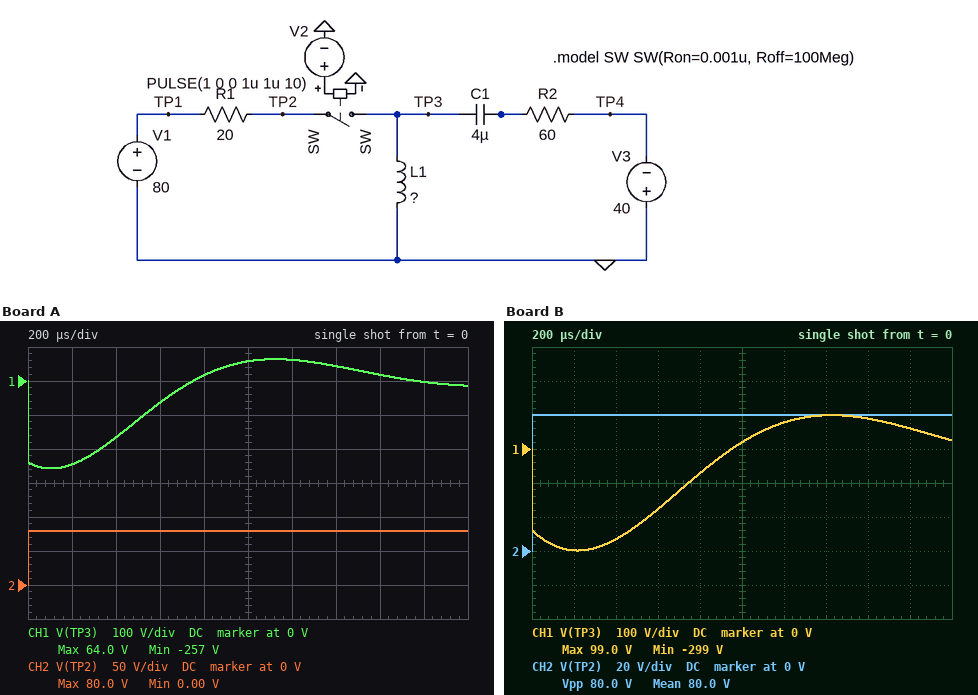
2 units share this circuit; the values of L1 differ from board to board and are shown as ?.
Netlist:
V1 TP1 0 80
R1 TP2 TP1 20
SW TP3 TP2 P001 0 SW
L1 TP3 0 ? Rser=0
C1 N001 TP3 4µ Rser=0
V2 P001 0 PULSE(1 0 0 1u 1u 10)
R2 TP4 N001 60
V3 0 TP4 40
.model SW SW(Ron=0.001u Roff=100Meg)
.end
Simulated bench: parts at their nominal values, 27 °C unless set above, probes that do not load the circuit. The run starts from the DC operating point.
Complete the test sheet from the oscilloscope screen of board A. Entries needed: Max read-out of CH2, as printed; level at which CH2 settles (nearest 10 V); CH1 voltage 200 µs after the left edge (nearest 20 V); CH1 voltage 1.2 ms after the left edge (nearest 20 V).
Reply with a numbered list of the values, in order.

1. 80.0 V
2. 80 V
3. -240 V
4. 60 V
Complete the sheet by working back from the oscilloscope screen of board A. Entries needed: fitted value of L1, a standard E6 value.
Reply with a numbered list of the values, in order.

1. 22 mH
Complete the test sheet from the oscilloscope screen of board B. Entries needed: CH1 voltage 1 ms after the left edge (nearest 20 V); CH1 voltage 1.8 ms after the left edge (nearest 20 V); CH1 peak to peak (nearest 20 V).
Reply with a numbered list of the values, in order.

1. 20 V
2. 60 V
3. 400 V
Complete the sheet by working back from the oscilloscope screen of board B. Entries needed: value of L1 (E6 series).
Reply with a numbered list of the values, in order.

1. 33 mH
